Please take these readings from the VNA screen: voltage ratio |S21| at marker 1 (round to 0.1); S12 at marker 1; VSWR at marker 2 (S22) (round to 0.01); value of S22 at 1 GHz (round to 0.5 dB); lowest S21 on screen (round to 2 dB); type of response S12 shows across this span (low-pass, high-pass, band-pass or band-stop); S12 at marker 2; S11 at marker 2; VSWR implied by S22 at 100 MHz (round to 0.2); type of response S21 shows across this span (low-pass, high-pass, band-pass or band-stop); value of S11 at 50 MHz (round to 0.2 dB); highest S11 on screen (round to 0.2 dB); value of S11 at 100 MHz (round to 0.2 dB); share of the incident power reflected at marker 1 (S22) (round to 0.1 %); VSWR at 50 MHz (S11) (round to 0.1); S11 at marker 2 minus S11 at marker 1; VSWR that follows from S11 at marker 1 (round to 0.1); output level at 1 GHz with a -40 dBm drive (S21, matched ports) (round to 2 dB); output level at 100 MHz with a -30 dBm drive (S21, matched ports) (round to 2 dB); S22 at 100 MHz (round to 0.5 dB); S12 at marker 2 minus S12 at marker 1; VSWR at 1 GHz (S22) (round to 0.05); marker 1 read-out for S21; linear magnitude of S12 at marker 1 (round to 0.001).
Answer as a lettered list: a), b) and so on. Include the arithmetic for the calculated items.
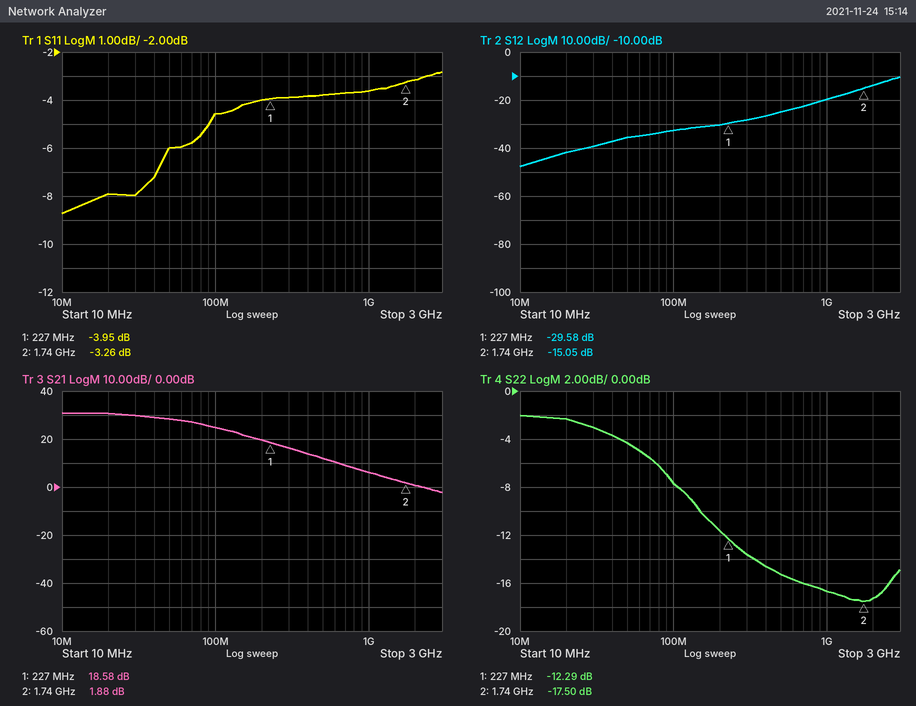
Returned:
a) 10^(18.58/20) ≈ 8.5
b) -29.58 dB
c) (1 + 0.1334)/(1 − 0.1334) ≈ 1.31
d) -16.5 dB
e) -2 dB
f) high-pass
g) -15.05 dB
h) -3.26 dB
i) |Γ| = 10^(-7.5/20) = 0.4217; VSWR = (1 + 0.4217)/(1 − 0.4217) ≈ 2.46, so 2.4 to the nearest 0.2
j) low-pass
k) -6.0 dB
l) -2.8 dB
m) -4.6 dB
n) 10^(-12.29/10) ≈ 5.9 %
o) |Γ| = 10^(-6/20) = 0.5012; VSWR = (1 + 0.5012)/(1 − 0.5012) ≈ 3.0
p) -3.26 − (-3.95) = 0.69 dB
q) (1 + 0.6346)/(1 − 0.6346) ≈ 4.5
r) -40 dBm + (6 dB) = -34 dBm
s) -30 dBm + (24 dB) = -6 dBm
t) -7.5 dB
u) -15.05 − (-29.58) = 14.53 dB
v) |Γ| = 10^(-16.5/20) = 0.1496; VSWR = (1 + 0.1496)/(1 − 0.1496) ≈ 1.35
w) 18.58 dB
x) 10^(-29.58/20) ≈ 0.033
